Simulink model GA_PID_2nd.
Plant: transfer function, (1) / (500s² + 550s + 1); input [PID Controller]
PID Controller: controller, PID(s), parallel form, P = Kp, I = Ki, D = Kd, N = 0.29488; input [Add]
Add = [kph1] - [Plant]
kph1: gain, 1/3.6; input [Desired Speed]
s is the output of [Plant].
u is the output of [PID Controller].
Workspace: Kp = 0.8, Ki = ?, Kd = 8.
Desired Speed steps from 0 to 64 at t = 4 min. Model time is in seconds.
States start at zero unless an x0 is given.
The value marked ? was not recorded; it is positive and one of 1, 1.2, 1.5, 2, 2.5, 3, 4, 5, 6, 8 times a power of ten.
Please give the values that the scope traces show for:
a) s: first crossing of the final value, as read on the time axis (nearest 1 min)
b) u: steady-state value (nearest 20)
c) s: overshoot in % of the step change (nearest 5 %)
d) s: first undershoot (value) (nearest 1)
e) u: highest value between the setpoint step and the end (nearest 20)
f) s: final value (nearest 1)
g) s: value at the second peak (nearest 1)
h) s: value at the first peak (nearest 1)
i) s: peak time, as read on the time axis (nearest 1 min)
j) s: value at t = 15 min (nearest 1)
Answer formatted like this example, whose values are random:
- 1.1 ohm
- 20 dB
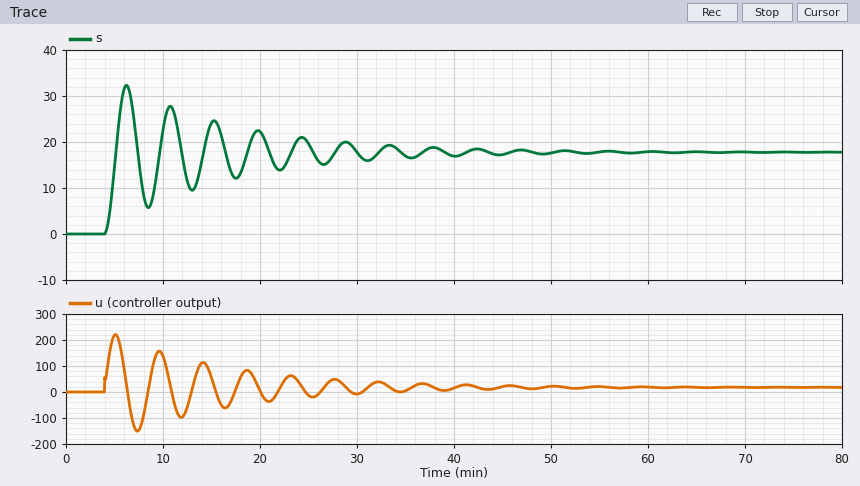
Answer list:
- 5 min
- 20
- 80 %
- 6
- 220
- 18
- 28
- 32
- 6 min
- 24
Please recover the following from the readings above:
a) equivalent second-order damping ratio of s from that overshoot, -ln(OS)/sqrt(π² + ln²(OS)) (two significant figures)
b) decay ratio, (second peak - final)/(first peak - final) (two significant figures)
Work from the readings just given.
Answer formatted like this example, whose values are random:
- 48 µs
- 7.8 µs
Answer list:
- 0.071
- 0.71
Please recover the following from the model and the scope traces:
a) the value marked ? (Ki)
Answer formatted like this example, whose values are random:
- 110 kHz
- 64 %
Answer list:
- 0.3
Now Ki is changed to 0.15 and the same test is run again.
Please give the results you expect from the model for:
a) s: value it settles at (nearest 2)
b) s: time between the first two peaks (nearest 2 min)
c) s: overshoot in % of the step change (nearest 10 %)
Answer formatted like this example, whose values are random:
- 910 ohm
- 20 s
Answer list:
- 18
- 6 min
- 70 %
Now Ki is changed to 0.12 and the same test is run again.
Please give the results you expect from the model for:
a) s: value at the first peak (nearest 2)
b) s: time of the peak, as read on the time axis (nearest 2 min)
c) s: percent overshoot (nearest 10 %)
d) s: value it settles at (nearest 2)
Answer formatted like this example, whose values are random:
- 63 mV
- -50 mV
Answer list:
- 30
- 8 min
- 70 %
- 18
